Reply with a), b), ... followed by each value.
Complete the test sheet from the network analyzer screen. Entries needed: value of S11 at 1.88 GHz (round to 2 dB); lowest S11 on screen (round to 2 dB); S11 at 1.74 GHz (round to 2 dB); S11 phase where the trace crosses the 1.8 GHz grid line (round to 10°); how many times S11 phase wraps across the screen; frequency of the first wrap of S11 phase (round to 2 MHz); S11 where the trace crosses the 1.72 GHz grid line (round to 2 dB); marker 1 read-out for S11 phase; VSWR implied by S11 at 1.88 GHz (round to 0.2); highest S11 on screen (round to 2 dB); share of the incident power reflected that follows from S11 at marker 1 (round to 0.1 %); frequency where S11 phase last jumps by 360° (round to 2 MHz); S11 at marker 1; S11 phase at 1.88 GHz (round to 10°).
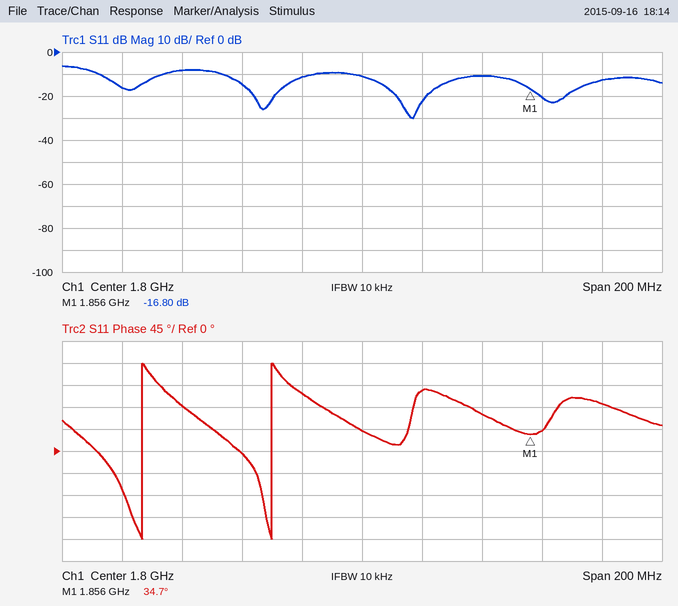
a) -12 dB
b) -30 dB
c) -8 dB
d) 40°
e) 2
f) 1.726 GHz
g) -16 dB
h) 34.7°
i) 1.6
j) -6 dB
k) 2.1 %
l) 1.770 GHz
m) -16.80 dB
n) 100°
